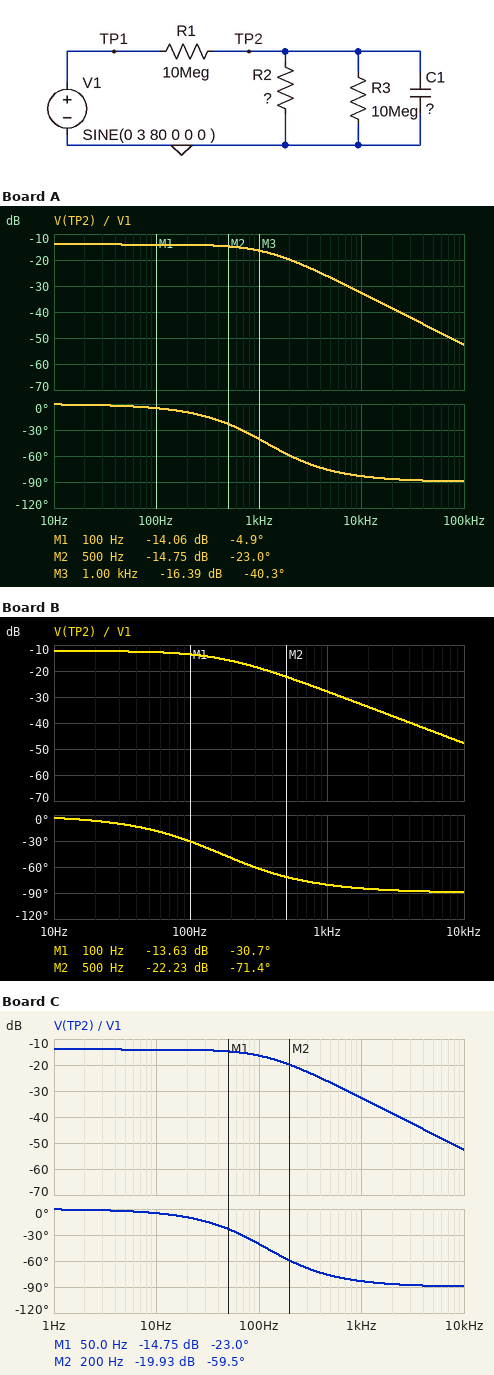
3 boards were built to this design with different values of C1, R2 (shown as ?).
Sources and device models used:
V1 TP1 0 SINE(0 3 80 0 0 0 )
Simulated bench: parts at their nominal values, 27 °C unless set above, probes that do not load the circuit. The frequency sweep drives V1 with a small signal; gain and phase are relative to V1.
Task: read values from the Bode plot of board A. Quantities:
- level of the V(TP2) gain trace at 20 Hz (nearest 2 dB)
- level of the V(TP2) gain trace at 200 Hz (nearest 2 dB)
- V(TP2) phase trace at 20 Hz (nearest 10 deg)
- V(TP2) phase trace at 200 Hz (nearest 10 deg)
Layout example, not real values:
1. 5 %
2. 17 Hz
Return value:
1. -14 dB
2. -14 dB
3. 0 deg
4. -10 deg
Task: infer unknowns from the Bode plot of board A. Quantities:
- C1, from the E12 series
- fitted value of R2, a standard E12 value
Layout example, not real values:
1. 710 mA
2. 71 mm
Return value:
1. 68 pF
2. 3.3 MΩ
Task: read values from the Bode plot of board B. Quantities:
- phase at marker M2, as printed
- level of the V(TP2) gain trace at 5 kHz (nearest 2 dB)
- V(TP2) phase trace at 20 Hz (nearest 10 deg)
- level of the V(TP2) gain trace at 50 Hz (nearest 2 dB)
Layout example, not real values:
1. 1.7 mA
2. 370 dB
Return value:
1. -71.4 deg
2. -42 dB
3. -10 deg
4. -12 dB
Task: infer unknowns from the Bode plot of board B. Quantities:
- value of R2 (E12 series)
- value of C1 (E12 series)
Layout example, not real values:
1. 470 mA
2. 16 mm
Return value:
1. 4.7 MΩ
2. 390 pF
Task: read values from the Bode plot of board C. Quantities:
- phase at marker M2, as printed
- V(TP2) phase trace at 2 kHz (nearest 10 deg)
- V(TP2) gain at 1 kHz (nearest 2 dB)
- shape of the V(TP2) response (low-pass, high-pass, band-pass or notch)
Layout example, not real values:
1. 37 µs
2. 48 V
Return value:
1. -59.5 deg
2. -90 deg
3. -32 dB
4. low-pass
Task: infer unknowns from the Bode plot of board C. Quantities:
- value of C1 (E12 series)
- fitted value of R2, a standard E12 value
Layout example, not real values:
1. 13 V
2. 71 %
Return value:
1. 680 pF
2. 3.3 MΩ
